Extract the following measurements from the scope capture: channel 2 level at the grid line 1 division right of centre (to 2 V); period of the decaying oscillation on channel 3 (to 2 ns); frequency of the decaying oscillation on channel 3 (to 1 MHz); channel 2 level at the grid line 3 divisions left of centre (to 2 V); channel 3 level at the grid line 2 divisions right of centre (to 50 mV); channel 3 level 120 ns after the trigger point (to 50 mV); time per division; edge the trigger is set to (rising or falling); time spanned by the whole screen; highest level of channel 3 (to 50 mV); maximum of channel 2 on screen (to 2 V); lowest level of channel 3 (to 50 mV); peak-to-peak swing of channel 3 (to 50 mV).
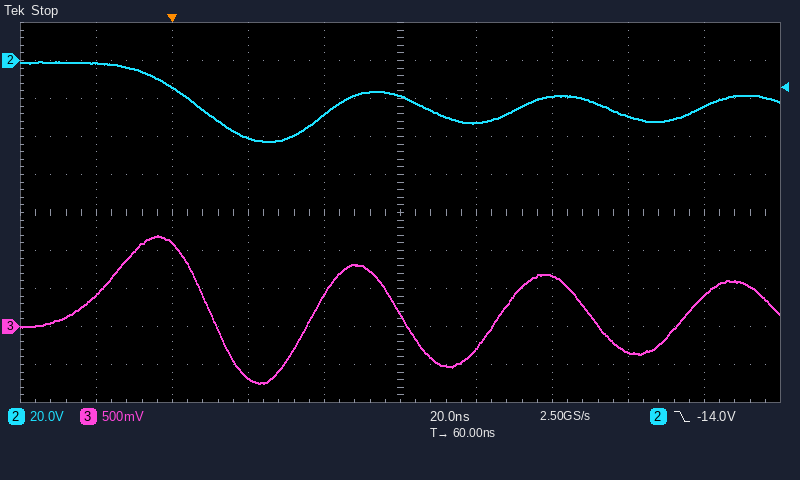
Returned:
-32 V
50 ns
20 MHz
-14 V
650 mV
-350 mV
20 ns
falling
200 ns
1.20 V
0 V
-750 mV
1.95 V
